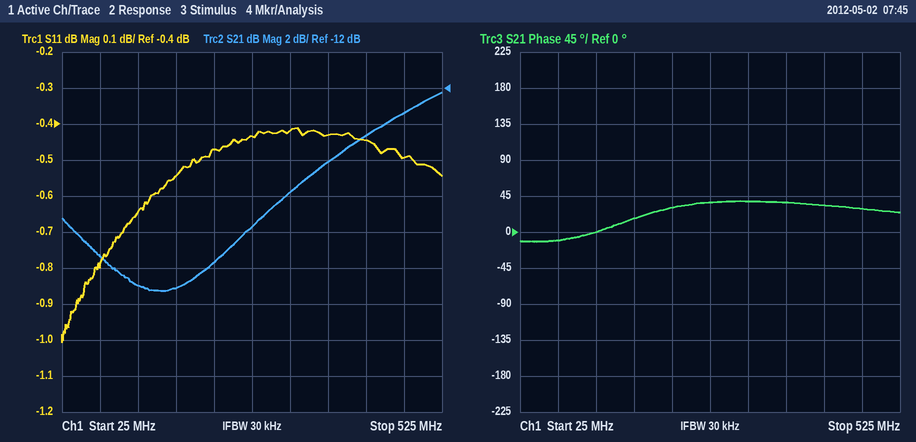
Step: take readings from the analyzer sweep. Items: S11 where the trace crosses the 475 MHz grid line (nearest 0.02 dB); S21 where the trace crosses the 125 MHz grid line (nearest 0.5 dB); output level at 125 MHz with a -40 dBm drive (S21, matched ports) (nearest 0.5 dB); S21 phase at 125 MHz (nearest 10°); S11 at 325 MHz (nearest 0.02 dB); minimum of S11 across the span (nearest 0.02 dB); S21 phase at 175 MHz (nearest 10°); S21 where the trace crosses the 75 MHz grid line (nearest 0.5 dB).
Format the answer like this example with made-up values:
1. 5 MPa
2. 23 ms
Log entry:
1. -0.50 dB
2. -23.0 dB
3. -63.0 dBm
4. 0°
5. -0.42 dB
6. -1.00 dB
7. 20°
8. -21.5 dB
